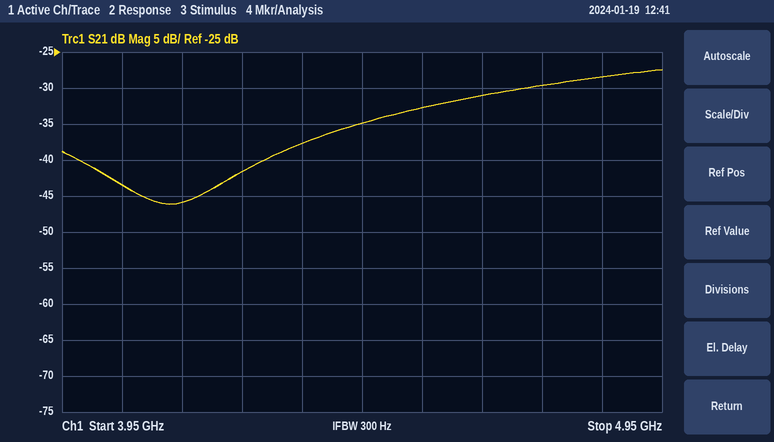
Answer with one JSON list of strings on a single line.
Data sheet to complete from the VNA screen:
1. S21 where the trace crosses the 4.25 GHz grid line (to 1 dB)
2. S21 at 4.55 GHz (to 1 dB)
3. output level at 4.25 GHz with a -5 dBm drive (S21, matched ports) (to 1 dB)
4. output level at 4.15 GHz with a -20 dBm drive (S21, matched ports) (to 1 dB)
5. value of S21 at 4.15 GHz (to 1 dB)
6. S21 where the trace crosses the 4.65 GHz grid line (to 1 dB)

["-42 dB", "-33 dB", "-47 dBm", "-66 dBm", "-46 dB", "-31 dB"]
